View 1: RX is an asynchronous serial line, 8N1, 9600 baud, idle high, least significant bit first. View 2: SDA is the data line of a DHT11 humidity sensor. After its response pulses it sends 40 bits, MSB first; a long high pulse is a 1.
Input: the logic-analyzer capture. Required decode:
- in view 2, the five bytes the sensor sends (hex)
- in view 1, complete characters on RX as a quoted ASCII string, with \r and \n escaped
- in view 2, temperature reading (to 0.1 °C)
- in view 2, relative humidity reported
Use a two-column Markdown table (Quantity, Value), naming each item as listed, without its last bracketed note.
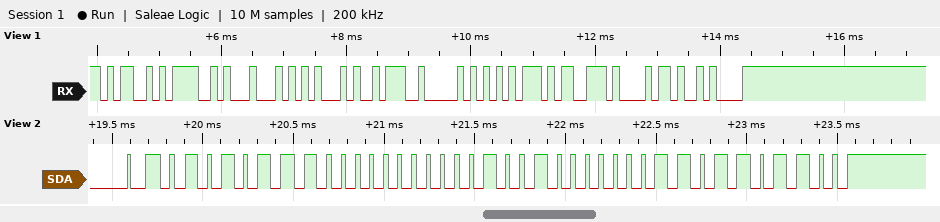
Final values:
| Quantity | Value |
|---|---|
| in view 2, the five bytes the sensor sends | 57 00 12 03 6C |
| in view 1, complete characters on RX as a quoted ASCII string, with \r and \n escaped | "MODE:Push\n" |
| in view 2, temperature reading | 18.3 °C |
| in view 2, relative humidity reported | 87 % |
